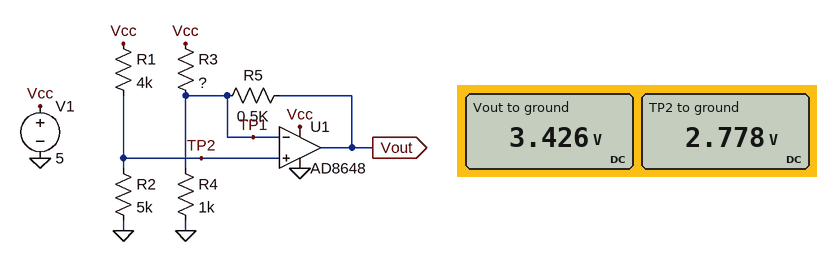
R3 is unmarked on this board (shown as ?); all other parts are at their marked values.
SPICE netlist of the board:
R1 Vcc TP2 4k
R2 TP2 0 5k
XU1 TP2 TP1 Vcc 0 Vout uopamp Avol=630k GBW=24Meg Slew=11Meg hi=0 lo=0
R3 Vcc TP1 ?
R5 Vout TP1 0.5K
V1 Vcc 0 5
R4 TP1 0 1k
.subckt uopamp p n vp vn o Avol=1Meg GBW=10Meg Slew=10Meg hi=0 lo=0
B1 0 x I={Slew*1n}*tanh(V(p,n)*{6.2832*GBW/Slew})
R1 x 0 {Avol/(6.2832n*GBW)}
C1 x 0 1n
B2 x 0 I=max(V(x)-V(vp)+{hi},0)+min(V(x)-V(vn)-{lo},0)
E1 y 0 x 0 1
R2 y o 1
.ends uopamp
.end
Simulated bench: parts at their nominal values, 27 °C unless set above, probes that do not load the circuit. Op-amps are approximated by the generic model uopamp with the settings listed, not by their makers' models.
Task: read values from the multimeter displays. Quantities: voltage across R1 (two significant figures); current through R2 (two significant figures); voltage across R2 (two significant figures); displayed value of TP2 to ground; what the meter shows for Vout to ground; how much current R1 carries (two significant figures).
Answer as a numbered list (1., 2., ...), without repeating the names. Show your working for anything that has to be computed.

1. 5 V - 2.778 V = 2.2 V
2. (2.778 V) / 5 kΩ = 560 µA
3. 2.778 V = 2.8 V
4. 2.778 V
5. 3.426 V
6. (5 V - 2.778 V) / 4 kΩ = 560 µA
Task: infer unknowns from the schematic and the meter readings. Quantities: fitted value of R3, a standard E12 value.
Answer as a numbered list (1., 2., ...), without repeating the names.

1. 1.5 kΩ
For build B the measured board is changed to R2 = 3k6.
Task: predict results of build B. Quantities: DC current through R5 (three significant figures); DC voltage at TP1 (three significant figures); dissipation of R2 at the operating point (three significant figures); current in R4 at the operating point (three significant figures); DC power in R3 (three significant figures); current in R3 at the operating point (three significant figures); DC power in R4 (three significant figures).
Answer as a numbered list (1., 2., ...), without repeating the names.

1. 614 µA
2. 2.37 V
3. 1.56 mW
4. 2.37 mA
5. 4.62 mW
6. 1.75 mA
7. 5.61 mW
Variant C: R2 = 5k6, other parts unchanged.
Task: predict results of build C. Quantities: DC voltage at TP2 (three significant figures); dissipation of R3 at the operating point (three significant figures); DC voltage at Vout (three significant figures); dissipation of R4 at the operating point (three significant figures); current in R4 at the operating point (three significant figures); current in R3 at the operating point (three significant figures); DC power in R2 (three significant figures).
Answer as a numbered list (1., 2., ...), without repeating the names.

1. 2.92 V
2. 2.89 mW
3. 3.68 V
4. 8.51 mW
5. 2.92 mA
6. 1.39 mA
7. 1.52 mW
